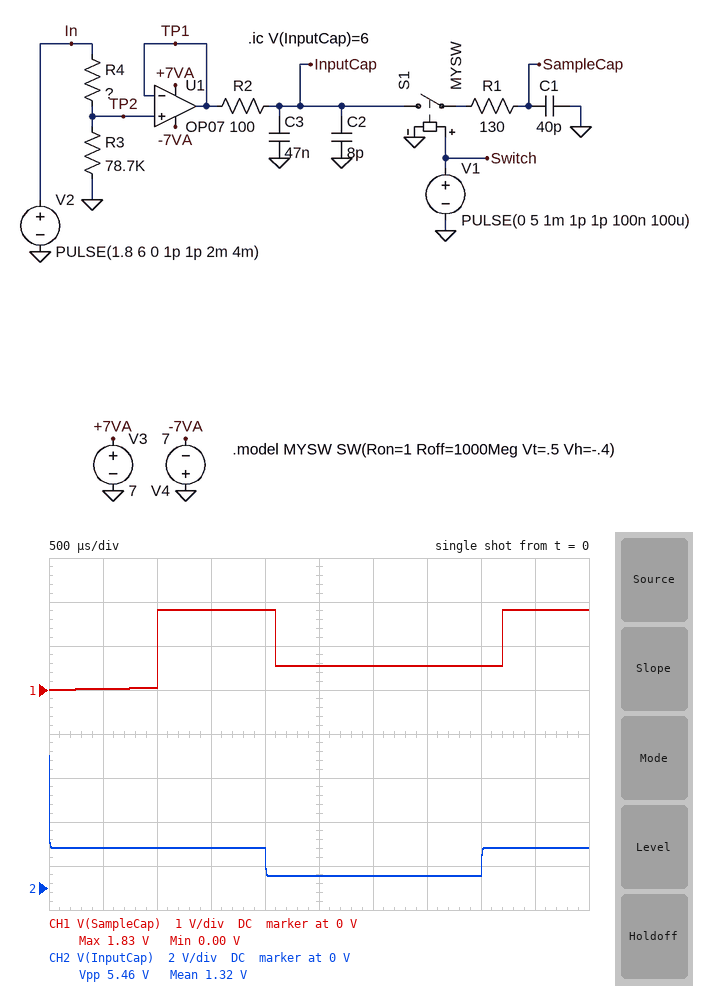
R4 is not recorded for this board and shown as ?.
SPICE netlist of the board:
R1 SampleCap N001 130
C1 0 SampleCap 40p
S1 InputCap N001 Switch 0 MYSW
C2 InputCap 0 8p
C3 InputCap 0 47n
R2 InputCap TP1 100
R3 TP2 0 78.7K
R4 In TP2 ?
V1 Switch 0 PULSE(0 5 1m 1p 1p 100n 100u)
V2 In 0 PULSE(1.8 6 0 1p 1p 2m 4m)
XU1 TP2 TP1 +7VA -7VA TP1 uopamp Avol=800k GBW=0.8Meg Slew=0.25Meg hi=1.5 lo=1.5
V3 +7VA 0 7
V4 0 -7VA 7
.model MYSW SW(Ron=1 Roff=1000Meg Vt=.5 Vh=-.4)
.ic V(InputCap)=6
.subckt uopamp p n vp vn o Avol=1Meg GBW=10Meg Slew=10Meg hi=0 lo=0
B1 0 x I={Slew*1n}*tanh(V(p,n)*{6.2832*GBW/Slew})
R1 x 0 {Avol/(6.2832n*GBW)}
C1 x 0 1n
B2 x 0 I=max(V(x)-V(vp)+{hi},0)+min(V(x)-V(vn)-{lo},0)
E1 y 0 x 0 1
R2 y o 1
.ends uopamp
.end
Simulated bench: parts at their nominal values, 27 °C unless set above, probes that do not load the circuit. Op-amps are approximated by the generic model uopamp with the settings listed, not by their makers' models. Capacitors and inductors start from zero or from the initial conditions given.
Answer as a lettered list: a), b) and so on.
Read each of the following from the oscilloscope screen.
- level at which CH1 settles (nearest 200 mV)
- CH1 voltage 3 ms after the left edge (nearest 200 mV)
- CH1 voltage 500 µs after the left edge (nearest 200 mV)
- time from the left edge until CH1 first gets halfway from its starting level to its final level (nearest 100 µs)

a) 1.8 V
b) 600 mV
c) 0 V
d) 1.0 ms
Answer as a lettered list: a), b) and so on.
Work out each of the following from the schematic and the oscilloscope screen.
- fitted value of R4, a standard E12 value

a) 180 kΩ
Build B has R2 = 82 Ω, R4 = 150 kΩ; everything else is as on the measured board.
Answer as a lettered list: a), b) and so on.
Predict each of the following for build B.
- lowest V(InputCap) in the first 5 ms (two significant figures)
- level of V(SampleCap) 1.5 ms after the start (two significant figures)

a) 620 mV
b) 2.1 V
